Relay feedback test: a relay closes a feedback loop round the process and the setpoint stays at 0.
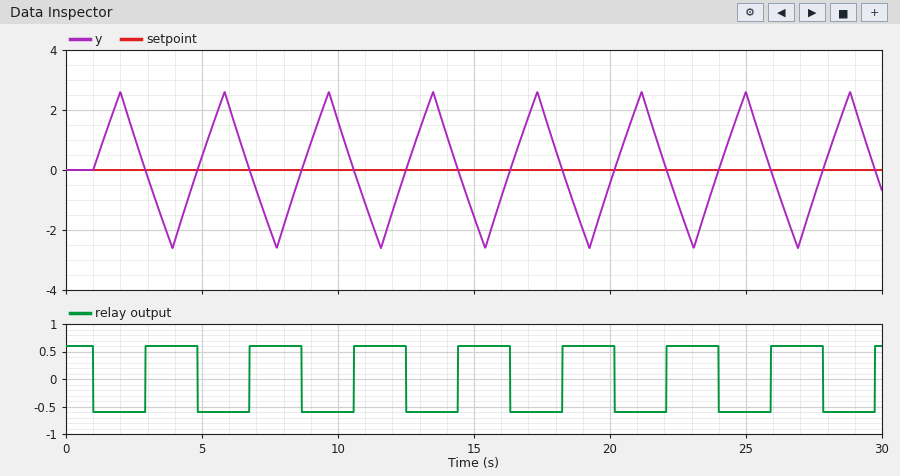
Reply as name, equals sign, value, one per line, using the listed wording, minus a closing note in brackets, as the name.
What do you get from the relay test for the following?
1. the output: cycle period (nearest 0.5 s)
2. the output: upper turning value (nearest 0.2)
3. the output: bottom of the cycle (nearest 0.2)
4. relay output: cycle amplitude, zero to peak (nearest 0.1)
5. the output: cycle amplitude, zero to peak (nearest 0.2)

the output: cycle period = 4.0 s
the output: upper turning value = 2.6
the output: bottom of the cycle = -2.6
relay output: cycle amplitude, zero to peak = 0.6
the output: cycle amplitude, zero to peak = 2.6
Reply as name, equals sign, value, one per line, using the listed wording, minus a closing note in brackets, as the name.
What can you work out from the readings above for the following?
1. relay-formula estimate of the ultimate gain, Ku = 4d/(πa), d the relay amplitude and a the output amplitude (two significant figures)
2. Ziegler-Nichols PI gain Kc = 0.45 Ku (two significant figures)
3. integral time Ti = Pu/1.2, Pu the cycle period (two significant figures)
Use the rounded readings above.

relay-formula estimate of the ultimate gain, Ku = 4d/(πa), d the relay amplitude and a the output amplitude = 0.29
Ziegler-Nichols PI gain Kc = 0.45 Ku = 0.13
integral time Ti = Pu/1.2, Pu the cycle period = 3.3 s
